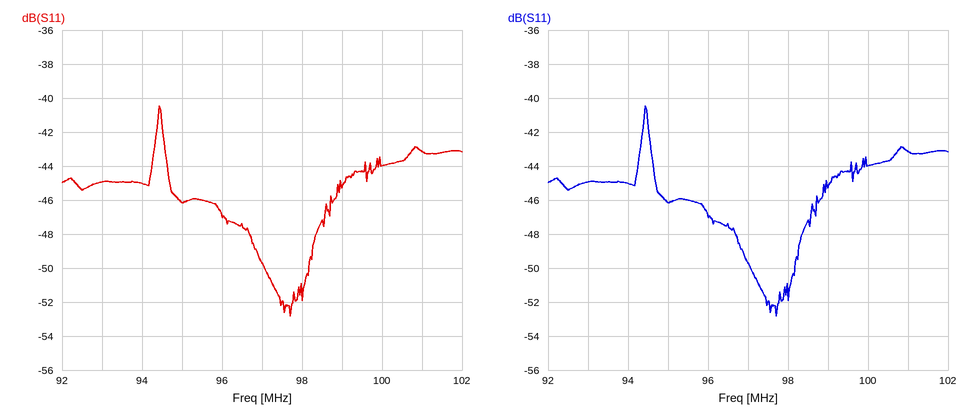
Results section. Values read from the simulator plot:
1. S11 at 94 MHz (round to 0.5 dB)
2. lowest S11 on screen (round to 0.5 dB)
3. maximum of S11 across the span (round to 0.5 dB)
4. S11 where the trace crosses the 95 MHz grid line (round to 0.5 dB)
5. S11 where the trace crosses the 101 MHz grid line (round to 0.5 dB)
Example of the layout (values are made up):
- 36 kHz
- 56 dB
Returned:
- -45.0 dB
- -53.0 dB
- -40.5 dB
- -46.0 dB
- -43.0 dB
